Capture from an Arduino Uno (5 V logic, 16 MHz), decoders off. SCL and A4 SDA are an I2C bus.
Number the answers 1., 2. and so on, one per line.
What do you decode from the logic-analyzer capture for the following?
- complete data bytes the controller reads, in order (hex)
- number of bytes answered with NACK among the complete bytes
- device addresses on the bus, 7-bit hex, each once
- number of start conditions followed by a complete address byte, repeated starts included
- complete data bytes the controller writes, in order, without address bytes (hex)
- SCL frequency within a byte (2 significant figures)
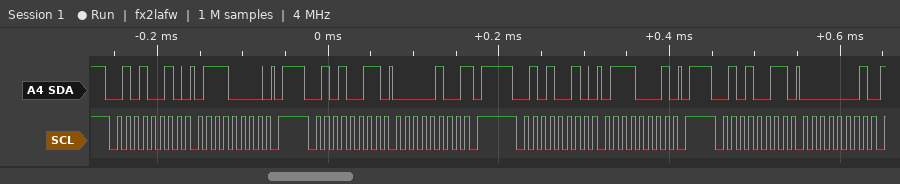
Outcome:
1. 04 01
2. 1
3. 0x29
4. 4
5. 70 71
6. 100 kHz
